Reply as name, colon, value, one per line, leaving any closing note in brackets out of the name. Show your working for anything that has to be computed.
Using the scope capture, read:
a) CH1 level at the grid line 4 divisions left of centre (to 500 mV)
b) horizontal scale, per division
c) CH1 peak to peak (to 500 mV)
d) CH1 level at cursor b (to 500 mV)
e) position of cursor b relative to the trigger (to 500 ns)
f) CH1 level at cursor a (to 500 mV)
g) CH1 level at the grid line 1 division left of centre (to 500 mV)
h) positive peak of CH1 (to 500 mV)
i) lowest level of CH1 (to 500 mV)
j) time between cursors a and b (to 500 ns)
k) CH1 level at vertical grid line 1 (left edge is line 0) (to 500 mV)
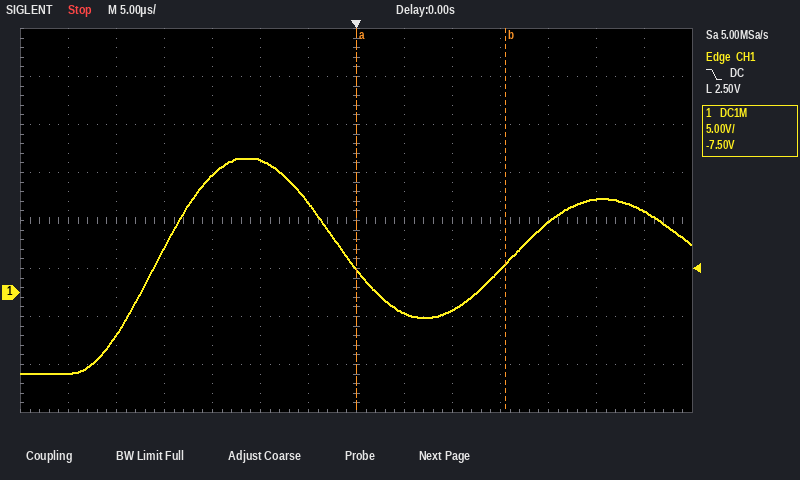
CH1 level at the grid line 4 divisions left of centre: 4.5 V
horizontal scale, per division: 5 µs
CH1 peak to peak: 14.0 V − (-8.5 V) = 22.5 V
CH1 level at cursor b: 3.0 V
position of cursor b relative to the trigger: +15.5 µs
CH1 level at cursor a: 2.5 V
CH1 level at the grid line 1 division left of centre: 9.5 V
positive peak of CH1: 14.0 V
lowest level of CH1: -8.5 V
time between cursors a and b: 15.5 µs
CH1 level at vertical grid line 1 (left edge is line 0): -8.5 V
